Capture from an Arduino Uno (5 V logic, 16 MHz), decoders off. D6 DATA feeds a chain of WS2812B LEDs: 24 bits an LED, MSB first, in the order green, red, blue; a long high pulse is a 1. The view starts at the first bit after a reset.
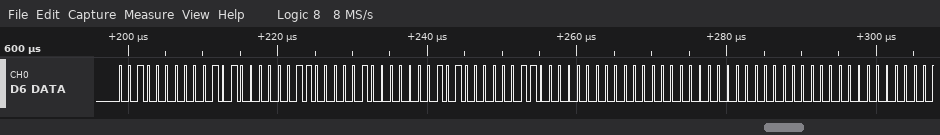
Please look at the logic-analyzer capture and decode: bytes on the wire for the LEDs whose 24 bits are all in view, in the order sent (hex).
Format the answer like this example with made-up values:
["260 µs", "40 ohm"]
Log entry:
["20 28 18 20 28 18 00 00 00"]
